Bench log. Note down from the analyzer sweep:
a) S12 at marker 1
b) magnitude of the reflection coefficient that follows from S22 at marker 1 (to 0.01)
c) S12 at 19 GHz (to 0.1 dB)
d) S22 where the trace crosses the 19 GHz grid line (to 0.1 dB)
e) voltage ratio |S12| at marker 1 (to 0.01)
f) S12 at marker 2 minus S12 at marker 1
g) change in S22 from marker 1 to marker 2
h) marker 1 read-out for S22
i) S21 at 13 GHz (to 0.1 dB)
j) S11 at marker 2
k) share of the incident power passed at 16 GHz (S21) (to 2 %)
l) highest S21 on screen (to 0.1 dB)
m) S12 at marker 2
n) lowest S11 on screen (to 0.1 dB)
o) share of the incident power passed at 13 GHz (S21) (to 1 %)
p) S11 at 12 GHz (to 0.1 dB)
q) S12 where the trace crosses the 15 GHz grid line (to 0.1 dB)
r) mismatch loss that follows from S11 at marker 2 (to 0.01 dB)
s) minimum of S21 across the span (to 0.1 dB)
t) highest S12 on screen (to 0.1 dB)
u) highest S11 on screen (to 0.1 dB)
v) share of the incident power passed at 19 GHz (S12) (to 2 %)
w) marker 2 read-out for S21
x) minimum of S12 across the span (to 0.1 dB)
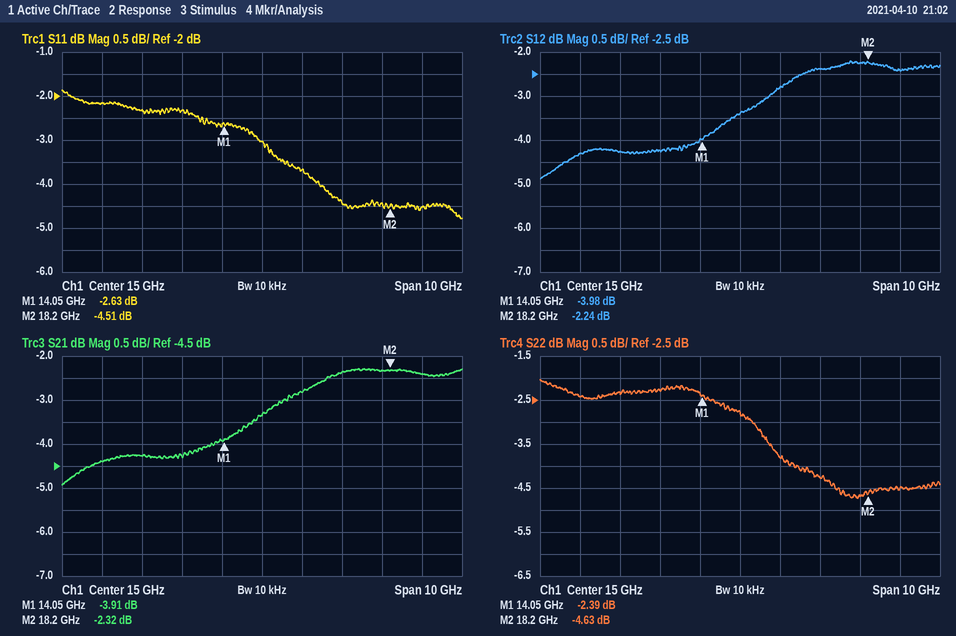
-3.98 dB
0.76
-2.4 dB
-4.5 dB
0.63
1.74 dB
-2.24 dB
-2.39 dB
-4.3 dB
-4.51 dB
52 %
-2.3 dB
-2.24 dB
-4.8 dB
37 %
-2.3 dB
-3.4 dB
1.90 dB
-4.9 dB
-2.2 dB
-1.9 dB
58 %
-2.32 dB
-4.9 dB
